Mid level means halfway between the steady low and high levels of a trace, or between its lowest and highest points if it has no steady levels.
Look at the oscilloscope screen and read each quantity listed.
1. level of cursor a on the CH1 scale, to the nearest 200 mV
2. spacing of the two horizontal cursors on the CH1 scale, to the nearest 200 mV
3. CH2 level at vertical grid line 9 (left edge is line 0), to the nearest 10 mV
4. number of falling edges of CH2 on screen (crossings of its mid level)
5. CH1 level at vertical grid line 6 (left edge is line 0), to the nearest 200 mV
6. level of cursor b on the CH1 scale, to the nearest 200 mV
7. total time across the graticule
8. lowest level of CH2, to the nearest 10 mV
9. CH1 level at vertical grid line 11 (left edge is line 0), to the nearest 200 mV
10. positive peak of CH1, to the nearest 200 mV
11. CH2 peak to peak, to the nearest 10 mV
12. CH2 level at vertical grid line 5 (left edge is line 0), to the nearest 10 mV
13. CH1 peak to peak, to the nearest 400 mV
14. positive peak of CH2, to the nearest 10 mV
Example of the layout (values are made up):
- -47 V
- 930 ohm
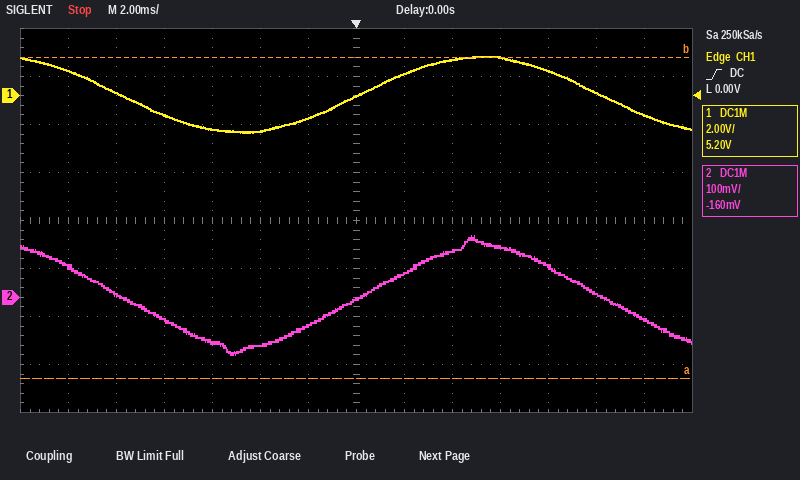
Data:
- -11.8 V
- 13.4 V
- 100 mV
- 2
- -1.0 V
- 1.6 V
- 28 ms
- -120 mV
- 1.0 V
- 1.6 V
- 250 mV
- -100 mV
- 3.2 V
- 130 mV
